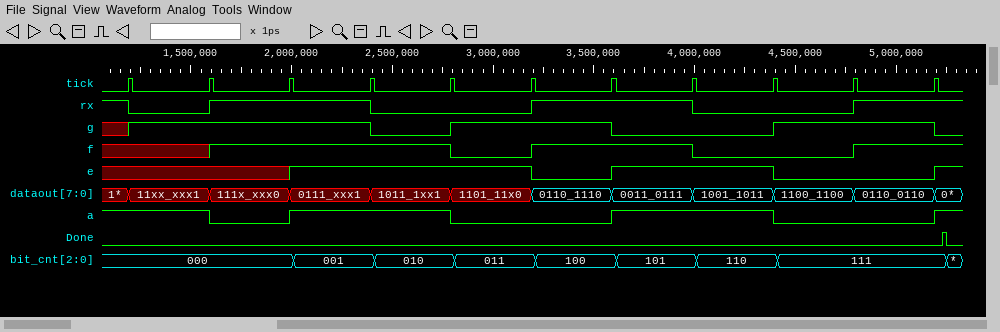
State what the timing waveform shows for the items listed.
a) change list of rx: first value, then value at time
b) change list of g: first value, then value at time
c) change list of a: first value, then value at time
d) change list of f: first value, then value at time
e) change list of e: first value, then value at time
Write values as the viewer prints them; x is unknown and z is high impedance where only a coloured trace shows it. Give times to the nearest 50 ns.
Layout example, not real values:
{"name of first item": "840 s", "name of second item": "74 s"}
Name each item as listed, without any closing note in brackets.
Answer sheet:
{"change list of rx: first value, then value at time": "1, 0 at 1200 ns, 1 at 1600 ns, 0 at 2400 ns, 1 at 3200 ns, 0 at 4000 ns, 1 at 4800 ns", "change list of g: first value, then value at time": "x, 1 at 1200 ns, 0 at 2400 ns, 1 at 2800 ns, 0 at 3600 ns, 1 at 4400 ns, 0 at 5200 ns", "change list of a: first value, then value at time": "1, 0 at 1600 ns, 1 at 2000 ns, 0 at 2800 ns, 1 at 3600 ns, 0 at 4400 ns, 1 at 5200 ns", "change list of f: first value, then value at time": "x, 1 at 1600 ns, 0 at 2800 ns, 1 at 3200 ns, 0 at 4000 ns, 1 at 4800 ns", "change list of e: first value, then value at time": "x, 1 at 2000 ns, 0 at 3200 ns, 1 at 3600 ns, 0 at 4400 ns, 1 at 5200 ns"}
